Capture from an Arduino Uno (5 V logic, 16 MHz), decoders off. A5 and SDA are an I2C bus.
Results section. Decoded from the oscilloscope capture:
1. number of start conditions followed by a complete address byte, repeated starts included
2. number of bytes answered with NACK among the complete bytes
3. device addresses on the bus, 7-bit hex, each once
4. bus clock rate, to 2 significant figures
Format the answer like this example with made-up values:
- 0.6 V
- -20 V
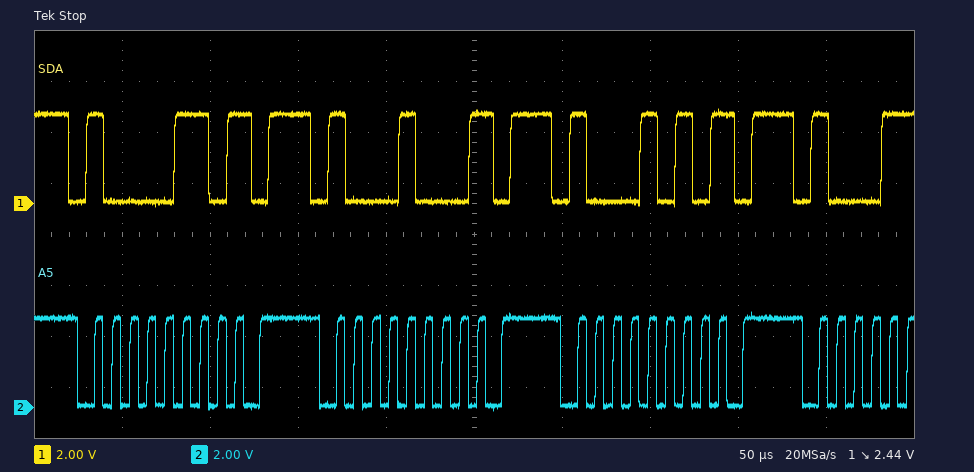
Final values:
- 3
- 3
- 0x43 0x44 0x45
- 100 kHz
